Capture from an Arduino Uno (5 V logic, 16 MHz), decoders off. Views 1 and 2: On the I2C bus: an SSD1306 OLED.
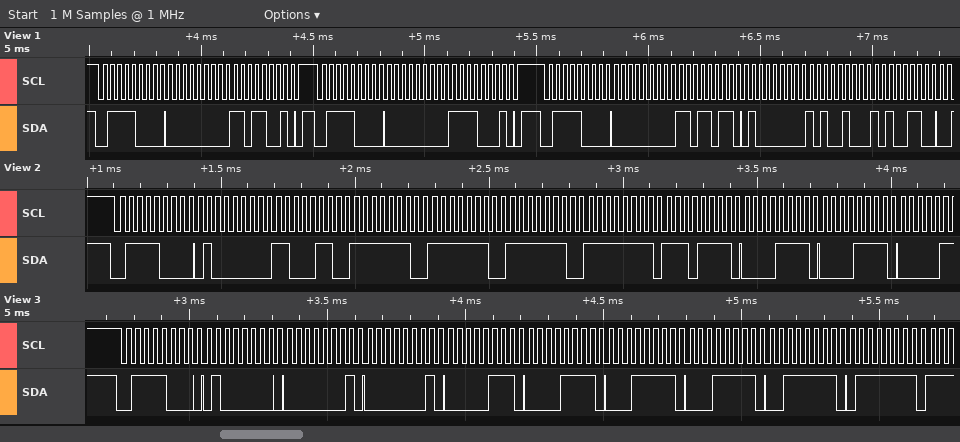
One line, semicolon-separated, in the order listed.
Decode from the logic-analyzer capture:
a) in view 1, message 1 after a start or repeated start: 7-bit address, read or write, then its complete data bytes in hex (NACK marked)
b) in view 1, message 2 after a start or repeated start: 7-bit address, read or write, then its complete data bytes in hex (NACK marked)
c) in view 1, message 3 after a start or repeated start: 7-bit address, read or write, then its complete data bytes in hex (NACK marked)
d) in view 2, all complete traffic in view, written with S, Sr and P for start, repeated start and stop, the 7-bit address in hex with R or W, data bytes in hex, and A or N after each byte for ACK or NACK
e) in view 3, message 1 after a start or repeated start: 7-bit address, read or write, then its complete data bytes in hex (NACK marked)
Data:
0x3C write: 00 D9; 0x3C write: 00 F1; 0x3C write: 00 DB 40 A4 A6; S 3CW A 40 A C6 A FE A FE A FE A FF A EF A 0F A 0F A; 0x3C write: 40 01 01 07 0F 1F 1F 3F 7F
